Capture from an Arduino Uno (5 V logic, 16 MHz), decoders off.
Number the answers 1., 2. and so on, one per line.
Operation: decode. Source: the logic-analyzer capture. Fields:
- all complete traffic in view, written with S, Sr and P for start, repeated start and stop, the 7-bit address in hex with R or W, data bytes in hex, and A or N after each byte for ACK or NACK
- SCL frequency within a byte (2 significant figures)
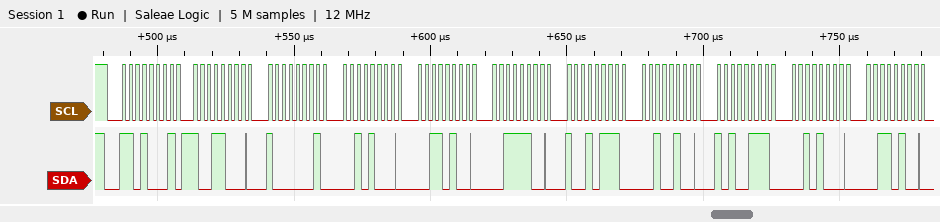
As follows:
1. S 68R A 98 A 81 A 28 A 34 A 3C A 97 A 24 A A7 A 28 A 34 A
2. 400 kHz
